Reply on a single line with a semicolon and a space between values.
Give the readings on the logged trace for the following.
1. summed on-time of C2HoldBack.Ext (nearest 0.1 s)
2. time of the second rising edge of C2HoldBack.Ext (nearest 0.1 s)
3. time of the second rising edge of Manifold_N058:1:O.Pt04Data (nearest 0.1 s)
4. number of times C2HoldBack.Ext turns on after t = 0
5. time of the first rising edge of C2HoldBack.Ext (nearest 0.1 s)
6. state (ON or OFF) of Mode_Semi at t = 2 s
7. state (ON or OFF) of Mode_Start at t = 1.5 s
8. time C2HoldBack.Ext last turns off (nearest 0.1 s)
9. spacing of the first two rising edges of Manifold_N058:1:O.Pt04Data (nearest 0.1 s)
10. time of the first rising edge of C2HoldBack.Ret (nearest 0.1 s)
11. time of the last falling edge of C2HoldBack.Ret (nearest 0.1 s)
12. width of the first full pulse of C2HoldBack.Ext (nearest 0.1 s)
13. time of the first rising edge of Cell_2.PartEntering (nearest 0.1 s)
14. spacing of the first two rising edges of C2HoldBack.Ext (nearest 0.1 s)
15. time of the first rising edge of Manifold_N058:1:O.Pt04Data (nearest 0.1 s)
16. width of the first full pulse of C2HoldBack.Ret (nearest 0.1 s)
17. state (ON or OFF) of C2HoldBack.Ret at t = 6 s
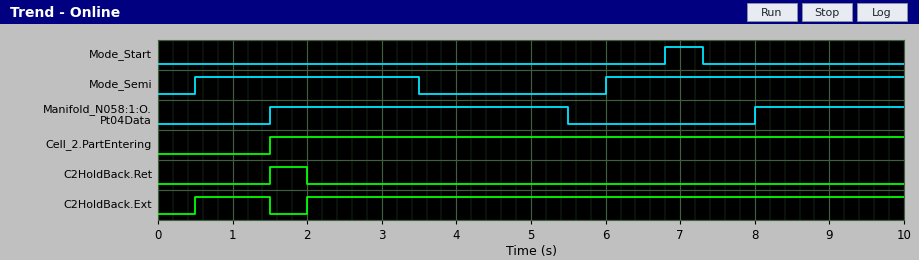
9.0 s; 2.0 s; 8.0 s; 2; 0.5 s; ON; OFF; 1.5 s; 6.5 s; 1.5 s; 2.0 s; 1.0 s; 1.5 s; 1.5 s; 1.5 s; 0.5 s; OFF
